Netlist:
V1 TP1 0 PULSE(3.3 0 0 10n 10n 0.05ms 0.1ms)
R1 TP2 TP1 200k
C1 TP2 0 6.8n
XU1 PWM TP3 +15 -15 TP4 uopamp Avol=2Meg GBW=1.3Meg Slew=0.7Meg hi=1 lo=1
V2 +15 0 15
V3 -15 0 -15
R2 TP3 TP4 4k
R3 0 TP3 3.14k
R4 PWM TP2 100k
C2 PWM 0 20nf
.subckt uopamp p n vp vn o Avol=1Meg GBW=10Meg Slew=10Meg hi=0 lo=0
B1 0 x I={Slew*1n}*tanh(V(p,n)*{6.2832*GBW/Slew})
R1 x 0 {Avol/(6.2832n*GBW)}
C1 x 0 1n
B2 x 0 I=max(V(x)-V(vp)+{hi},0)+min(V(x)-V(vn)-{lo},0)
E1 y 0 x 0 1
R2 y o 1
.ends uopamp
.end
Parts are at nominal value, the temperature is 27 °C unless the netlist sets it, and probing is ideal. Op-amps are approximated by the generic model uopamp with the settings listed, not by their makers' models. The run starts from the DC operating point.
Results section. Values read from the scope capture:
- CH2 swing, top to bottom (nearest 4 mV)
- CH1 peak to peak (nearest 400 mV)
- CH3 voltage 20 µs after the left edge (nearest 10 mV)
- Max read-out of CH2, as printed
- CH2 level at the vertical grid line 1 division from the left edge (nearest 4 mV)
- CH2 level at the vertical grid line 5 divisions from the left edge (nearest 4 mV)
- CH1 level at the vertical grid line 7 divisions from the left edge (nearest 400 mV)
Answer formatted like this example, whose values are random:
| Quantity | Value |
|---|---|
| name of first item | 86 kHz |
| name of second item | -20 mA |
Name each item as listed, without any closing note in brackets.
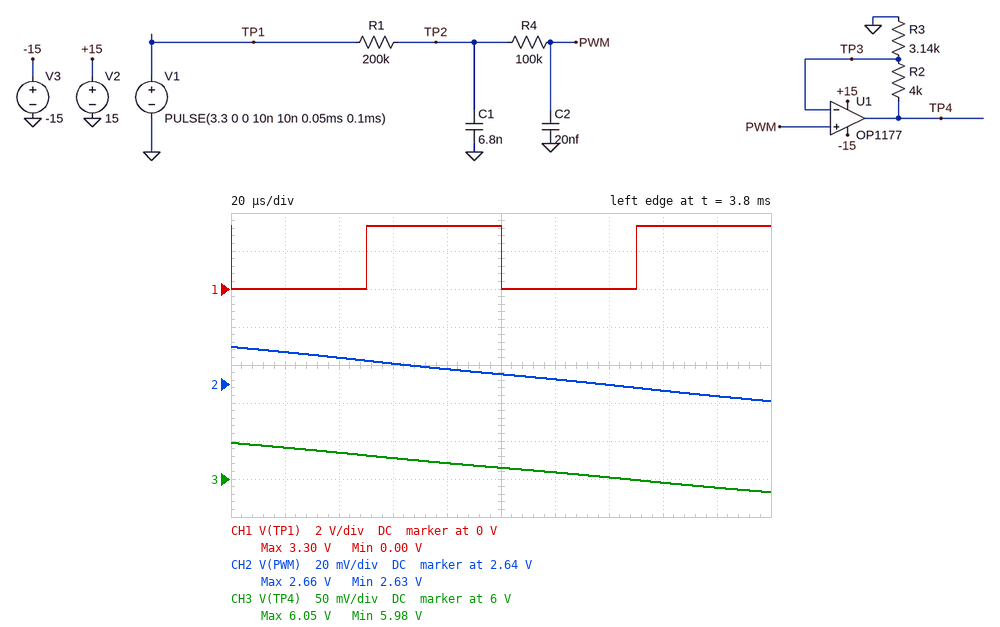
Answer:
| Quantity | Value |
|---|---|
| CH2 swing, top to bottom | 28 mV |
| CH1 peak to peak | 3.2 V |
| CH3 voltage 20 µs after the left edge | 6.04 V |
| Max read-out of CH2, as printed | 2.66 V |
| CH2 level at the vertical grid line 1 division from the left edge | 2.656 V |
| CH2 level at the vertical grid line 5 divisions from the left edge | 2.644 V |
| CH1 level at the vertical grid line 7 divisions from the left edge | 0 V |
